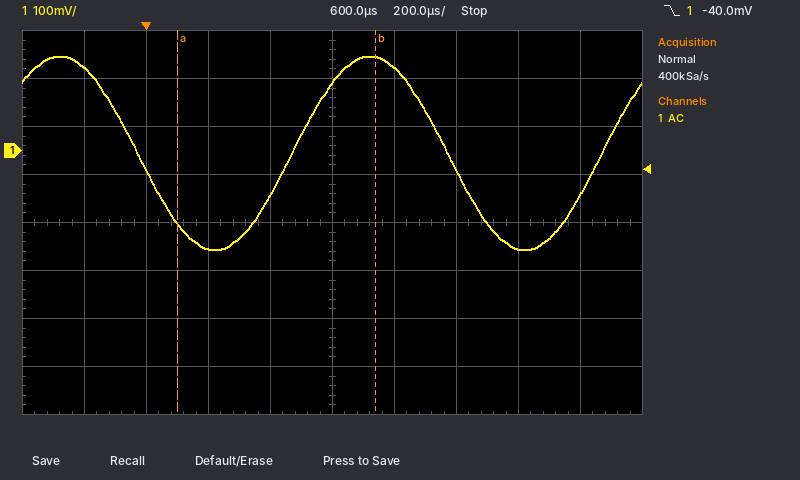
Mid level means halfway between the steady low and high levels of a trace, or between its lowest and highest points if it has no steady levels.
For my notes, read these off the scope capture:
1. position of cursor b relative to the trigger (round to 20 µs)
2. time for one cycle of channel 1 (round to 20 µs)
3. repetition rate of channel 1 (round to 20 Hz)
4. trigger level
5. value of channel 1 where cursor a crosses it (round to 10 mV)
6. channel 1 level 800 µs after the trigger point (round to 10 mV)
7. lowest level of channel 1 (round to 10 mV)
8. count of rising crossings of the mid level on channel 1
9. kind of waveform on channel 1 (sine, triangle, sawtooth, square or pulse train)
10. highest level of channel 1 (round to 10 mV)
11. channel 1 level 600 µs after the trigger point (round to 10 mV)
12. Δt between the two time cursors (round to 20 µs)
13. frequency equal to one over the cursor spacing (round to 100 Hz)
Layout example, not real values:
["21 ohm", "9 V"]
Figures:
["+740 µs", "1.00 ms", "1.00 kHz", "-40.0 mV", "-150 mV", "170 mV", "-210 mV", "2", "sine", "200 mV", "140 mV", "640 µs", "1.6 kHz"]
